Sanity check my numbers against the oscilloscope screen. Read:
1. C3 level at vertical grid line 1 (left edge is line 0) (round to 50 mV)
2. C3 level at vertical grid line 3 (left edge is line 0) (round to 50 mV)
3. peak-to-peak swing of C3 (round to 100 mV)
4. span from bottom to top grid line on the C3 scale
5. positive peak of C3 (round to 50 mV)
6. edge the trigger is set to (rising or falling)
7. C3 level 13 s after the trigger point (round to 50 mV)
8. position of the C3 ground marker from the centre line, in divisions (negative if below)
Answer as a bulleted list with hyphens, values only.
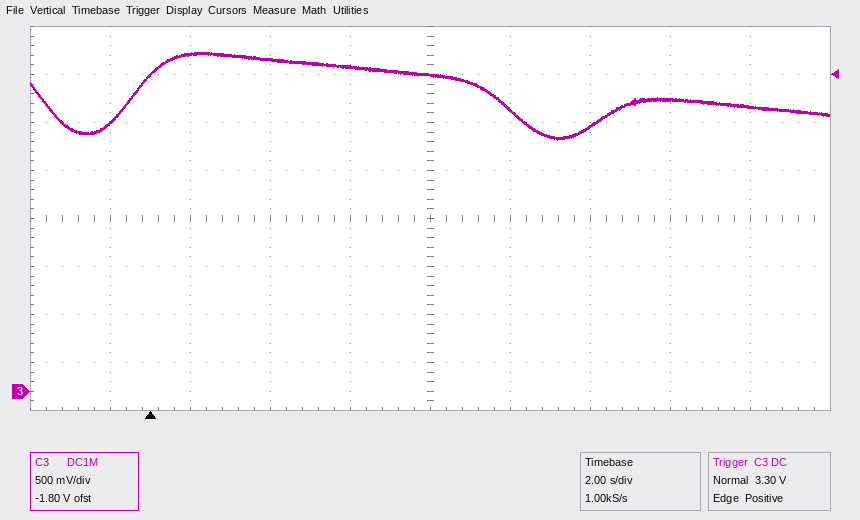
- 2.80 V
- 3.45 V
- 900 mV
- 4 V
- 3.55 V
- rising
- 3.05 V
- -3.6 div
